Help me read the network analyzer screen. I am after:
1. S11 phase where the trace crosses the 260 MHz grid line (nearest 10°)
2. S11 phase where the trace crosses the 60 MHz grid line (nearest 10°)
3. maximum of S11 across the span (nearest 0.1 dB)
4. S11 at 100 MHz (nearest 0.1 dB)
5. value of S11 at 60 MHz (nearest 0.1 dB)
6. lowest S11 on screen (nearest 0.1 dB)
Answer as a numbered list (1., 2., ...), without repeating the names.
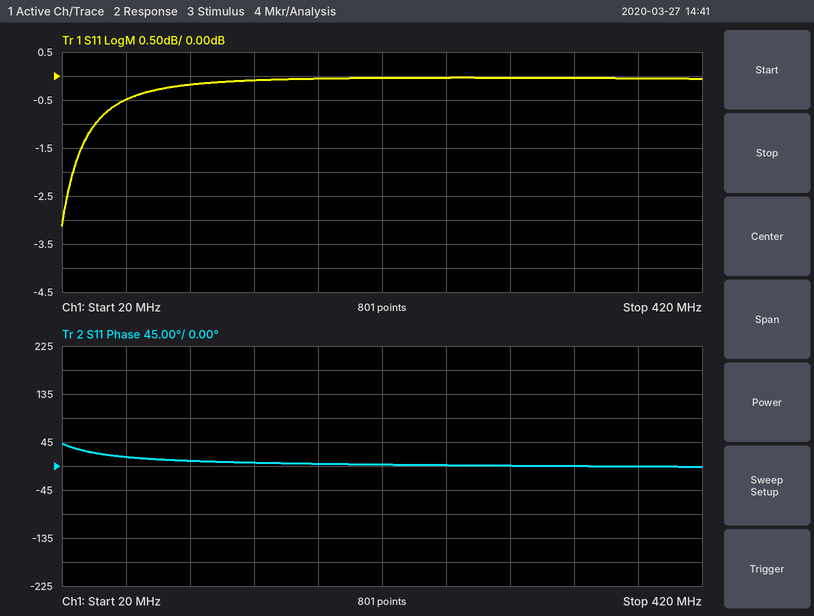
1. 0°
2. 20°
3. 0.0 dB
4. -0.2 dB
5. -0.5 dB
6. -3.1 dB
